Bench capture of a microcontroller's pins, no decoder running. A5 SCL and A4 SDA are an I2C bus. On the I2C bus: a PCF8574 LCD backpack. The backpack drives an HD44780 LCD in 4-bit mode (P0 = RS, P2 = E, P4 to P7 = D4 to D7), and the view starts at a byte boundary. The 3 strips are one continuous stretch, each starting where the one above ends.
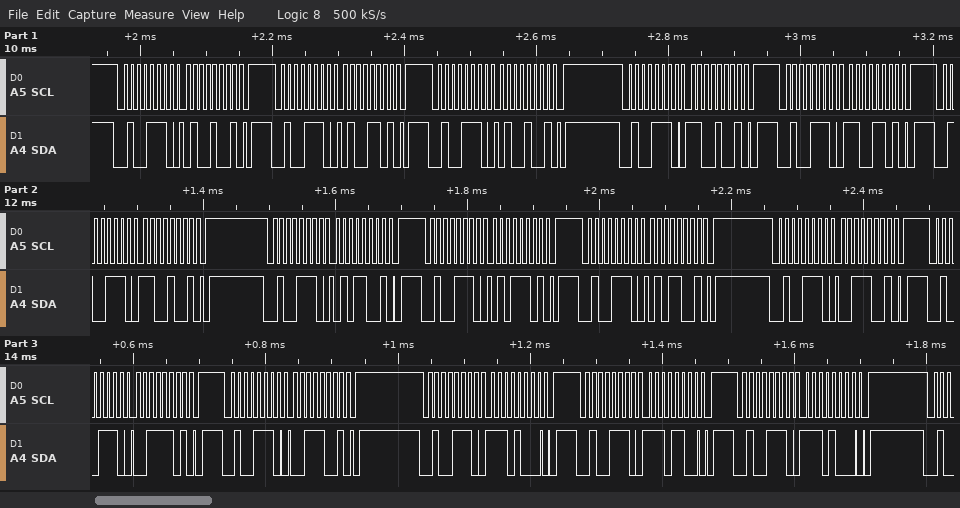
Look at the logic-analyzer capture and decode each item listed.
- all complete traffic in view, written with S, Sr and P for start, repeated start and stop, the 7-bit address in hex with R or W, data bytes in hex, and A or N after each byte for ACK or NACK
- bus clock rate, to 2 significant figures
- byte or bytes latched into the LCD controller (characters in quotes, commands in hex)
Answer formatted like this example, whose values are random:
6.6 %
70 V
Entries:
S 27W A 49 A P S 27W A 4D A P S 27W A 49 A P S 27W A C9 A P S 27W A CD A P S 27W A C9 A P S 27W A 59 A P S 27W A 5D A P S 27W A 59 A P S 27W A 39 A P S 27W A 3D A P S 27W A 39 A P S 27W A E8 A P S 27W A EC A P S 27W A E8 A P
100 kHz
'L' 'S'
